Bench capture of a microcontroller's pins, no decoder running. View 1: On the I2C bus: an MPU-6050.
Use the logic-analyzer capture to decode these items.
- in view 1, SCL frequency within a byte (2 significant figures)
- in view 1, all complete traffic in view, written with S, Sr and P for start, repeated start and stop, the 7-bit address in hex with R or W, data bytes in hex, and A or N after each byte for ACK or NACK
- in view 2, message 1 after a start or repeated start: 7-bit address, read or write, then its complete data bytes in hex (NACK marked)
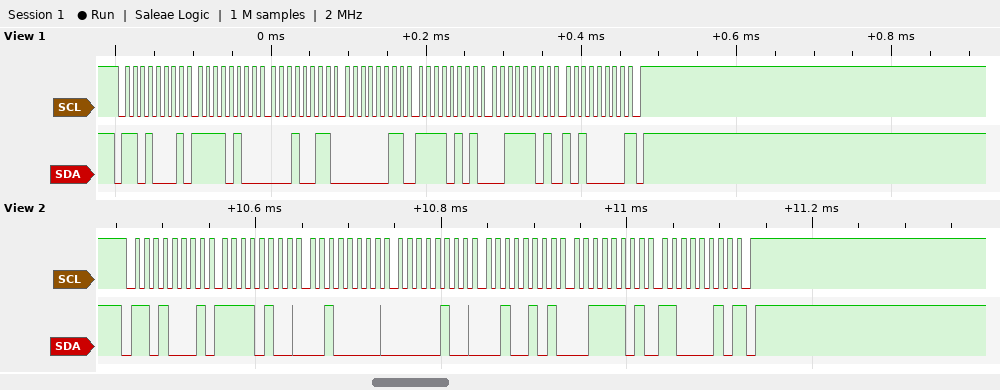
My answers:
100 kHz
S 68R A F4 A 13 A 03 A F5 A 3D A A0 N P
0x68 read: F4 20 04 25 3D C2 NACK
